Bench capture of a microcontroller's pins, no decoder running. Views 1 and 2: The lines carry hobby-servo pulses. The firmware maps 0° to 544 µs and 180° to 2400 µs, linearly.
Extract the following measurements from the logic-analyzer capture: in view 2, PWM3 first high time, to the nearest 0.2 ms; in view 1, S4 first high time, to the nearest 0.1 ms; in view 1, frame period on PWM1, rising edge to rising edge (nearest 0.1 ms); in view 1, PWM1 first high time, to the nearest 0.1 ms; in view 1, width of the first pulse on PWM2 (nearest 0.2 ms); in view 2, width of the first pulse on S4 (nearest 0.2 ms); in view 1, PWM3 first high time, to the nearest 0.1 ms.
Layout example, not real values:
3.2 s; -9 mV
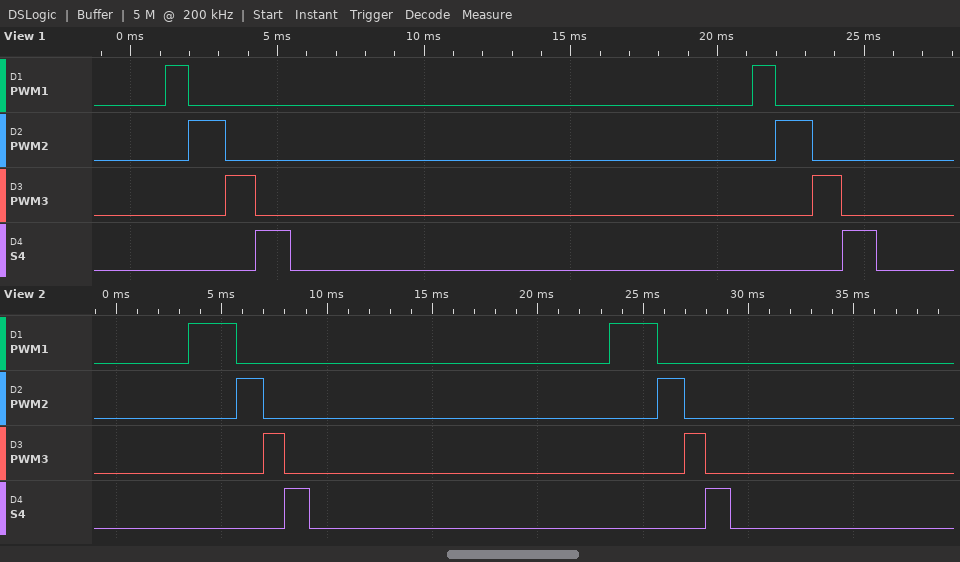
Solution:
1.0 ms; 1.2 ms; 20.0 ms; 0.8 ms; 1.2 ms; 1.2 ms; 1.0 ms
